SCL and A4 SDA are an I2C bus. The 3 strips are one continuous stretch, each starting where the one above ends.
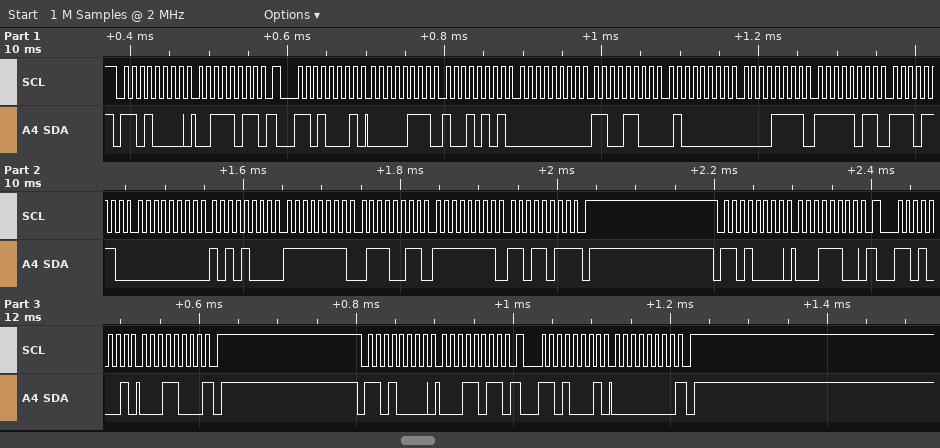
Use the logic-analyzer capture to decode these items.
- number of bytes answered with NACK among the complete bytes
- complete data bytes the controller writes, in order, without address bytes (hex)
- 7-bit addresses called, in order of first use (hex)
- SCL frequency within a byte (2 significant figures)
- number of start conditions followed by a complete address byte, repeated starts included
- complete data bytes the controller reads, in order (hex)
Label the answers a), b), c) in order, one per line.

a) 3
b) 3B 1C 1B
c) 0x68
d) 100 kHz
e) 6
f) 07 95 00 CC 40 0F FB EE 00 A8 FF 73 FF DB 18 00
